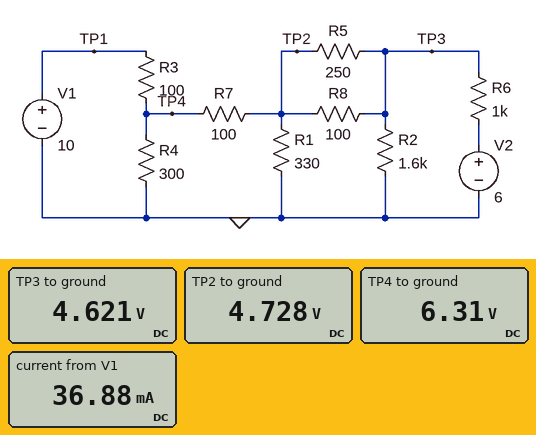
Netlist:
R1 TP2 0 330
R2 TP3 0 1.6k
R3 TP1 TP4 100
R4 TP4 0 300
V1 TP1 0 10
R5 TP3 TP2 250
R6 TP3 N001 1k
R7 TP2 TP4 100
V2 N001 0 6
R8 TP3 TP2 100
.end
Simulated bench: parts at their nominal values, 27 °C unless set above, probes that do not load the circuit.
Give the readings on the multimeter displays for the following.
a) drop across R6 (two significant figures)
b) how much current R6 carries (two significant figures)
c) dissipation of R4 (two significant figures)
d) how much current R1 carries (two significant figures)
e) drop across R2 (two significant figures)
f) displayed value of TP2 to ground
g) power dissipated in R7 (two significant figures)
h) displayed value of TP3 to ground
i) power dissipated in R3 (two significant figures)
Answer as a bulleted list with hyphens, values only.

- 1.4 V
- 1.4 mA
- 130 mW
- 14 mA
- 4.6 V
- 4.728 V
- 25 mW
- 4.621 V
- 140 mW
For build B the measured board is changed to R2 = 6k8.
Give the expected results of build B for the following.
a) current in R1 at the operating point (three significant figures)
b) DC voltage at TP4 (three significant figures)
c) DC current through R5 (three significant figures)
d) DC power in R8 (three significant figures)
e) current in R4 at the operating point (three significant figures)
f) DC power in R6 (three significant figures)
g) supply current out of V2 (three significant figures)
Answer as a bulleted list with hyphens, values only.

- 15.0 mA
- 6.40 V
- 89.1 µA
- 4.96 µW
- 21.3 mA
- 1.08 mW
- 1.04 mA
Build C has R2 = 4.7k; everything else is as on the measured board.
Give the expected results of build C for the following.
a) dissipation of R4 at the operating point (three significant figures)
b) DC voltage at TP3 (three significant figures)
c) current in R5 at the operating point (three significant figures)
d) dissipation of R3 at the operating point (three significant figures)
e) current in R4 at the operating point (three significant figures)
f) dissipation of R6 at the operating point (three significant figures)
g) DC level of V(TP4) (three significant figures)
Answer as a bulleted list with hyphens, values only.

- 136 mW
- 4.91 V
- 13.1 µA
- 130 mW
- 21.3 mA
- 1.19 mW
- 6.39 V
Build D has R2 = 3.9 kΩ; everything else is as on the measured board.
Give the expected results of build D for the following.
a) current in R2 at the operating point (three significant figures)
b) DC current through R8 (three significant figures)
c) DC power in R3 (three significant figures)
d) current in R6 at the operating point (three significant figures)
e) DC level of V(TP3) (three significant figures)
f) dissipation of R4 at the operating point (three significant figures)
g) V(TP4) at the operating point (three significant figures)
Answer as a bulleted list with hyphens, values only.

- 1.25 mA
- 91.3 µA
- 131 mW
- 1.12 mA
- 4.88 V
- 136 mW
- 6.38 V
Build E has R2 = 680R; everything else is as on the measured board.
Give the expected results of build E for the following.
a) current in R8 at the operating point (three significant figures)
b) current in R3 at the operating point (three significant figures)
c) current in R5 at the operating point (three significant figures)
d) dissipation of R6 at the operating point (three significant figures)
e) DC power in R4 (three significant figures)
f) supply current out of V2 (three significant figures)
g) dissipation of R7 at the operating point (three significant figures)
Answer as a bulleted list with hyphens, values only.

- 2.99 mA
- 38.2 mA
- 1.20 mA
- 3.52 mW
- 127 mW
- 1.88 mA
- 30.9 mW
